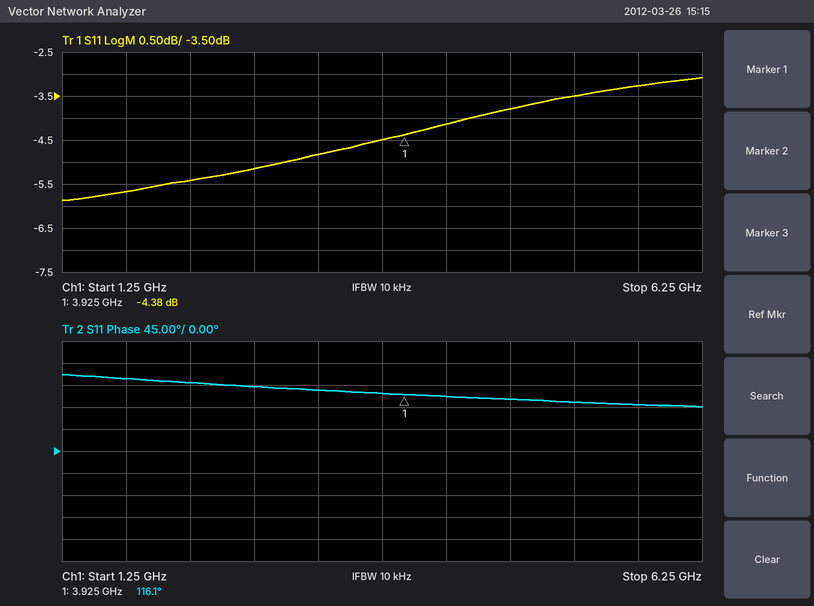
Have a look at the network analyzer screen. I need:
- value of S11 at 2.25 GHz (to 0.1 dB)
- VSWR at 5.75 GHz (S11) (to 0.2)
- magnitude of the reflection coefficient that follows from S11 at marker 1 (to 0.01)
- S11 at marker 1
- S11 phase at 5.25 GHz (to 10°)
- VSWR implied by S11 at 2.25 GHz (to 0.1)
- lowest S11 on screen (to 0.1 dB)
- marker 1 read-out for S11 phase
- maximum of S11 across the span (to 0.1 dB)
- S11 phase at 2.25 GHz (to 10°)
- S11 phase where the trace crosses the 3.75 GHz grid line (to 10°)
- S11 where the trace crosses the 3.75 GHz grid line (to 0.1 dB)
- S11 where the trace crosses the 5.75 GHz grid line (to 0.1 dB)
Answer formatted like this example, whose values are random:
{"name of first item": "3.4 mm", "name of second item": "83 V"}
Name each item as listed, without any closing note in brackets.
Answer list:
{"value of S11 at 2.25 GHz": "-5.4 dB", "VSWR at 5.75 GHz (S11)": "5.4", "magnitude of the reflection coefficient that follows from S11 at marker 1": "0.60", "S11 at marker 1": "-4.38 dB", "S11 phase at 5.25 GHz": "100°", "VSWR implied by S11 at 2.25 GHz": "3.3", "lowest S11 on screen": "-5.9 dB", "marker 1 read-out for S11 phase": "116.1°", "maximum of S11 across the span": "-3.1 dB", "S11 phase at 2.25 GHz": "140°", "S11 phase where the trace crosses the 3.75 GHz grid line": "120°", "S11 where the trace crosses the 3.75 GHz grid line": "-4.5 dB", "S11 where the trace crosses the 5.75 GHz grid line": "-3.3 dB"}
